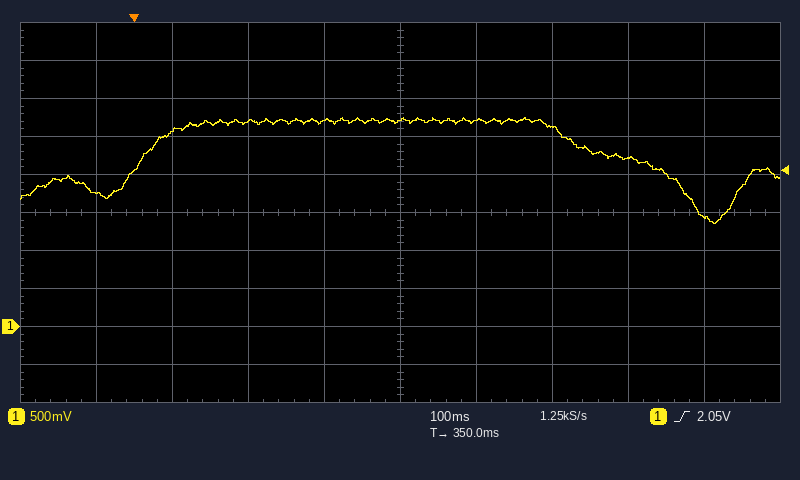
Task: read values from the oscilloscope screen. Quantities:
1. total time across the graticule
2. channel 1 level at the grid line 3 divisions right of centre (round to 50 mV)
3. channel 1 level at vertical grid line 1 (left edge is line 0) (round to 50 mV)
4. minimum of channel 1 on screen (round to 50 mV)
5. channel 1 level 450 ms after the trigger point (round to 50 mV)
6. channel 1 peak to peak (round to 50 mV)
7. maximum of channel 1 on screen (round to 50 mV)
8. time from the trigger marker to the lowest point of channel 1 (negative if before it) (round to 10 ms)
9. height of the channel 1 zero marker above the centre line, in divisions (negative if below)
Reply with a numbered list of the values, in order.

1. 1 s
2. 2.20 V
3. 1.75 V
4. 1.35 V
5. 2.70 V
6. 1.40 V
7. 2.75 V
8. +760 ms
9. -3.0 div
